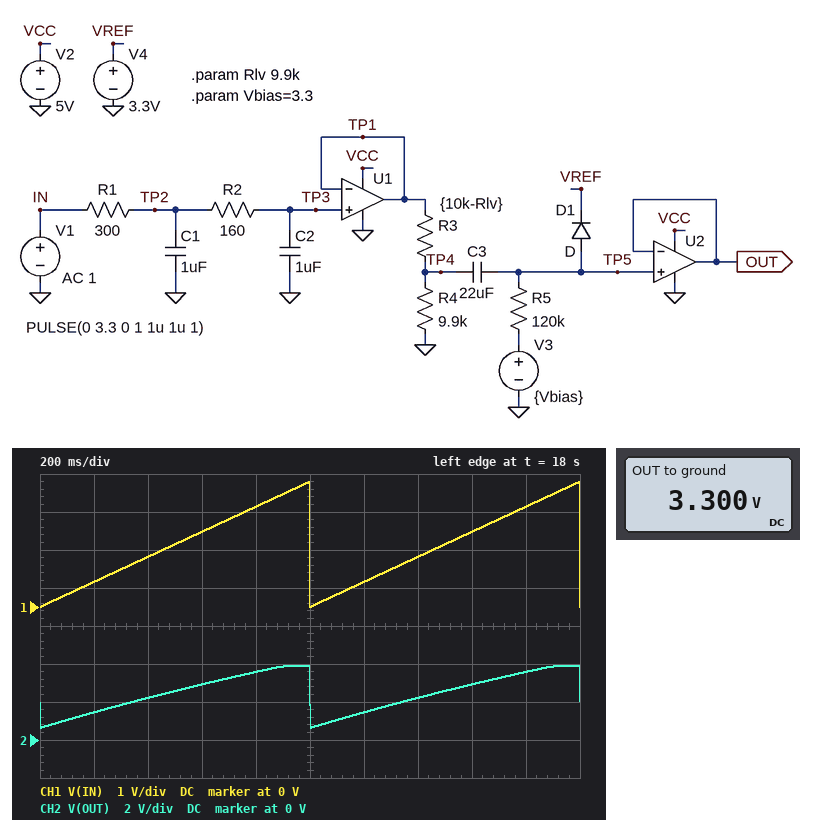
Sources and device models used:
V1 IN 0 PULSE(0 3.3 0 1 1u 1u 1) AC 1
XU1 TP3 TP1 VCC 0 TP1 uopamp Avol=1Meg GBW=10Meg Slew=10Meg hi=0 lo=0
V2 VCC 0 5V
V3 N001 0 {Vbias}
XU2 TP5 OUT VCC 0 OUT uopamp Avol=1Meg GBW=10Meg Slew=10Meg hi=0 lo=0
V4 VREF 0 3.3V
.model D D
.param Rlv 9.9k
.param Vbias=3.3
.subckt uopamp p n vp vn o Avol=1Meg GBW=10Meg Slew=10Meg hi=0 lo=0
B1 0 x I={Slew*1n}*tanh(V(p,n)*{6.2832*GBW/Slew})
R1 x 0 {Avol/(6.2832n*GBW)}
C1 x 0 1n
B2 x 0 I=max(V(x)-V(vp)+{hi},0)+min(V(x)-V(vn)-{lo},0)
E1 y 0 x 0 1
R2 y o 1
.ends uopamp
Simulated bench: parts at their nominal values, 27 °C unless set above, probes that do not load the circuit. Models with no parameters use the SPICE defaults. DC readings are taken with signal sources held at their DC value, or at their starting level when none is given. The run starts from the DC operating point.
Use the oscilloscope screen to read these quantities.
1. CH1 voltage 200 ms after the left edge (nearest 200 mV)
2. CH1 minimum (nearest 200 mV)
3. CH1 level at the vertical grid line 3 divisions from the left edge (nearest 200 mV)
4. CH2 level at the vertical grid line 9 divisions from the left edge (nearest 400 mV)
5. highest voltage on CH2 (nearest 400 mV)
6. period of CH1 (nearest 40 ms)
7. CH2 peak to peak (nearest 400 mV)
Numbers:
600 mV
0 V
2.0 V
3.6 V
4.0 V
1.00 s
3.2 V
